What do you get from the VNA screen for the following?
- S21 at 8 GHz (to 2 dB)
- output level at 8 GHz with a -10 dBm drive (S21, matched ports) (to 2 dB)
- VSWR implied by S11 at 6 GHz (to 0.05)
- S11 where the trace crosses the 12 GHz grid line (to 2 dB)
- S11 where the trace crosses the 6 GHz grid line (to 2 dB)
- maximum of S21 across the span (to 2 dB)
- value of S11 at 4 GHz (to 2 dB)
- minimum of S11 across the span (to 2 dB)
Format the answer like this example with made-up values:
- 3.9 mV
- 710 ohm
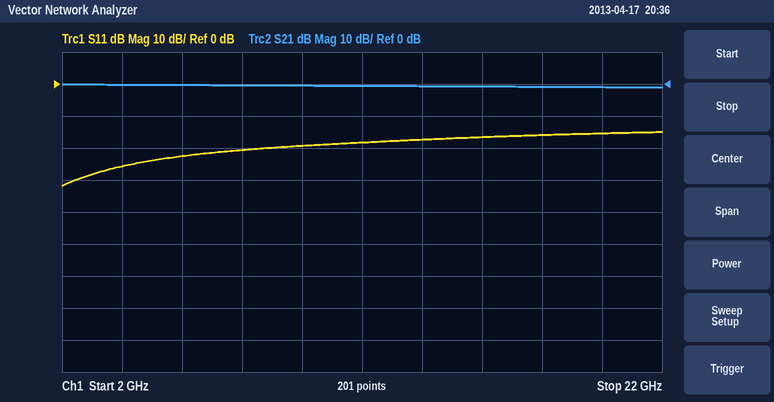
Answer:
- 0 dB
- -10 dBm
- 1.15
- -18 dB
- -22 dB
- 0 dB
- -26 dB
- -32 dB
